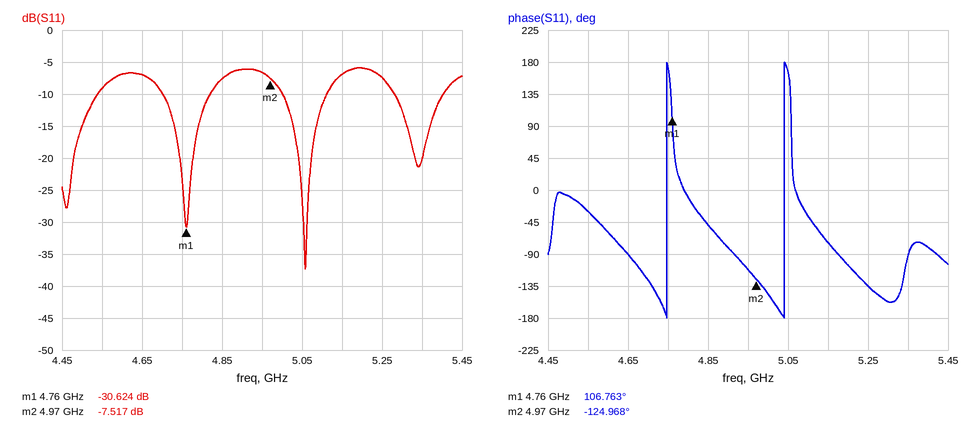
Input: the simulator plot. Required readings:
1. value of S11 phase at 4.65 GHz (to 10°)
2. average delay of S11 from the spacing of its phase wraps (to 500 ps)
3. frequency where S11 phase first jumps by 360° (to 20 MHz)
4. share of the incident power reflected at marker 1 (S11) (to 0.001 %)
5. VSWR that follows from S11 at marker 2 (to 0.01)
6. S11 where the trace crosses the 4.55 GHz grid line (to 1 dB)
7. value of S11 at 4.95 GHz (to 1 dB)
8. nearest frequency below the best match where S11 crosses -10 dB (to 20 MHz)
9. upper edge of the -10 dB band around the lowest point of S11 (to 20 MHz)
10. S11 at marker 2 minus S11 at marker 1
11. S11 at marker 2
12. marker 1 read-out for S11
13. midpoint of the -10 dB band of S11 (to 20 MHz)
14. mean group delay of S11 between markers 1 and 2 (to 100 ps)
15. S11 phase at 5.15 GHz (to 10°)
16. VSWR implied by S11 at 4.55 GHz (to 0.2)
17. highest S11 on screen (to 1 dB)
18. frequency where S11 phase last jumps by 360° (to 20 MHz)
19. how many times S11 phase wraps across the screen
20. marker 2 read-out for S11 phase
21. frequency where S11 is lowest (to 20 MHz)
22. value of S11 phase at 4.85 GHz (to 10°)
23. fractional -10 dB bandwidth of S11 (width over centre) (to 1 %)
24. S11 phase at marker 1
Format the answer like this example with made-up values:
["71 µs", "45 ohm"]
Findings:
["-90°", "3.5 ns", "4.74 GHz", "0.087 %", "2.45", "-9 dB", "-7 dB", "5.00 GHz", "5.12 GHz", "23.107 dB", "-7.517 dB", "-30.624 dB", "5.06 GHz", "3.1 ns", "-70°", "2.0", "-6 dB", "5.04 GHz", "2", "-124.968°", "5.06 GHz", "-50°", "2 %", "106.763°"]
